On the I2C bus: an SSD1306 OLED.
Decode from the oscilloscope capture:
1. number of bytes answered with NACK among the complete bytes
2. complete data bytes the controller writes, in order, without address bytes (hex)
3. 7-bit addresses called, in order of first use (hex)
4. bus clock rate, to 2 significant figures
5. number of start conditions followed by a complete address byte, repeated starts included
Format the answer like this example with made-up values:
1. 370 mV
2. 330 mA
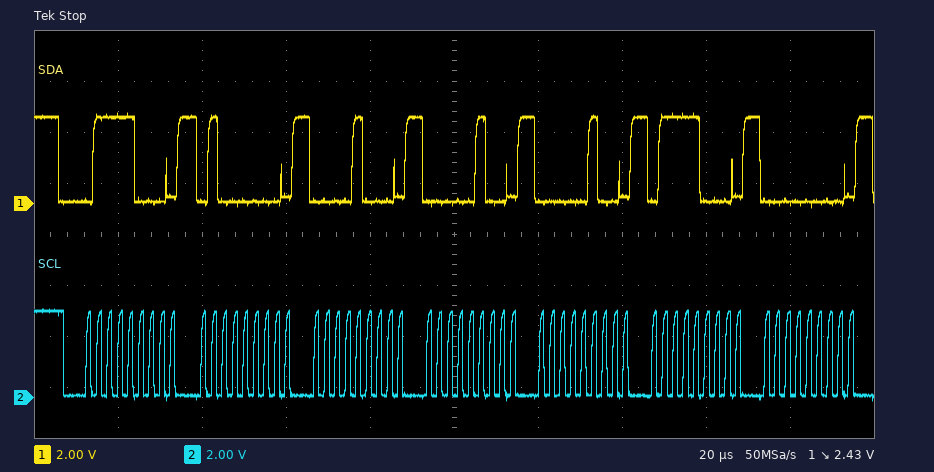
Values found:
1. 0
2. 40 08 04 04 78 00
3. 0x3C
4. 400 kHz
5. 1
